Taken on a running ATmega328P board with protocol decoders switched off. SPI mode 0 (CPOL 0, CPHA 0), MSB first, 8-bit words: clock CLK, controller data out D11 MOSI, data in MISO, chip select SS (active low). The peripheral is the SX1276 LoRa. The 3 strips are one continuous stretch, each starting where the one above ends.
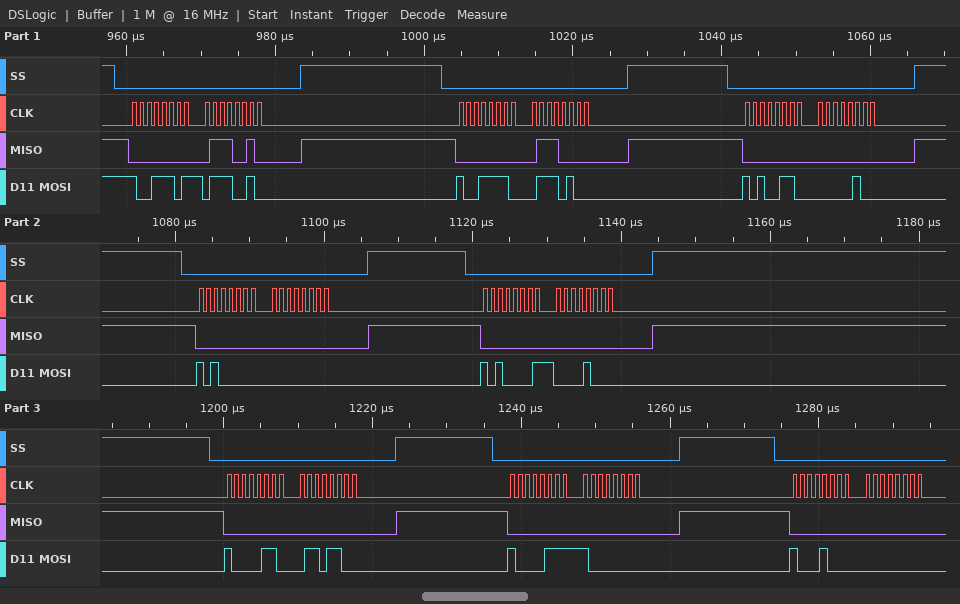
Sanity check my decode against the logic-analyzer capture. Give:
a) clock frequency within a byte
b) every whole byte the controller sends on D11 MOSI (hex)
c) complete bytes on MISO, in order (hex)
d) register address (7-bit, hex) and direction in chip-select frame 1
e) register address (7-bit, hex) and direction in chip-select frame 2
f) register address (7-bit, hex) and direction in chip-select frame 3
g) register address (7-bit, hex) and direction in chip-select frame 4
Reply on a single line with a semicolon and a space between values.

1 MHz; 9D 72 9E 74 A6 04 A0 00 A1 08 86 6C 87 80 88 00; 00 72 00 70 00 00 00 00 00 00 00 00 00 00 00 00; 0x1D write; 0x1E write; 0x26 write; 0x20 write
